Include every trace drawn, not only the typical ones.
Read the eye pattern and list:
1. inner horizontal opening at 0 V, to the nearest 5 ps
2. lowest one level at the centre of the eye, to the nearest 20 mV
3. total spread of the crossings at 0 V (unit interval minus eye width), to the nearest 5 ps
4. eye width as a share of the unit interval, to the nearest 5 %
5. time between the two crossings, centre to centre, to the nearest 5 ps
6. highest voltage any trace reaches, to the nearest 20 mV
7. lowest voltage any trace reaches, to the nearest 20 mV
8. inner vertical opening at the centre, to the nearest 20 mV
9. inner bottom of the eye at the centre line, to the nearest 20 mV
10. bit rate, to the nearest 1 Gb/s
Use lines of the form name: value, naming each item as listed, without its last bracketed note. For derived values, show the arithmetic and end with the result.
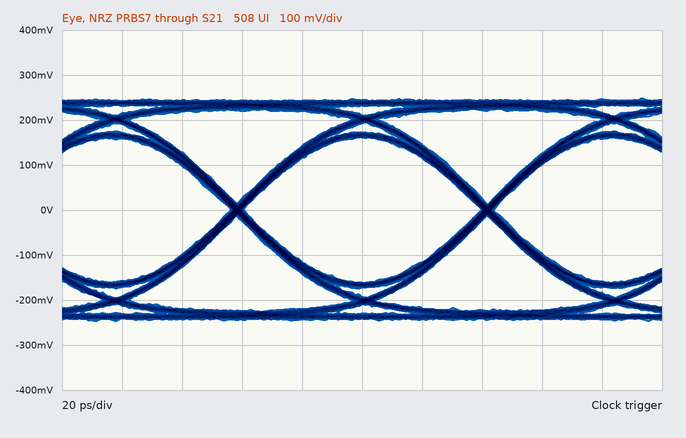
inner horizontal opening at 0 V, to the nearest 5 ps: 80 ps
lowest one level at the centre of the eye, to the nearest 20 mV: 160 mV
total spread of the crossings at 0 V (unit interval minus eye width), to the nearest 5 ps: 5 ps
eye width as a share of the unit interval, to the nearest 5 %: 80 ps / 85 ps ≈ 94.1 %, so 95 % to the nearest 5 %
time between the two crossings, centre to centre, to the nearest 5 ps: 85 ps
highest voltage any trace reaches, to the nearest 20 mV: 240 mV
lowest voltage any trace reaches, to the nearest 20 mV: -240 mV
inner vertical opening at the centre, to the nearest 20 mV: 320 mV
inner bottom of the eye at the centre line, to the nearest 20 mV: -160 mV
bit rate, to the nearest 1 Gb/s: 12 Gb/s
